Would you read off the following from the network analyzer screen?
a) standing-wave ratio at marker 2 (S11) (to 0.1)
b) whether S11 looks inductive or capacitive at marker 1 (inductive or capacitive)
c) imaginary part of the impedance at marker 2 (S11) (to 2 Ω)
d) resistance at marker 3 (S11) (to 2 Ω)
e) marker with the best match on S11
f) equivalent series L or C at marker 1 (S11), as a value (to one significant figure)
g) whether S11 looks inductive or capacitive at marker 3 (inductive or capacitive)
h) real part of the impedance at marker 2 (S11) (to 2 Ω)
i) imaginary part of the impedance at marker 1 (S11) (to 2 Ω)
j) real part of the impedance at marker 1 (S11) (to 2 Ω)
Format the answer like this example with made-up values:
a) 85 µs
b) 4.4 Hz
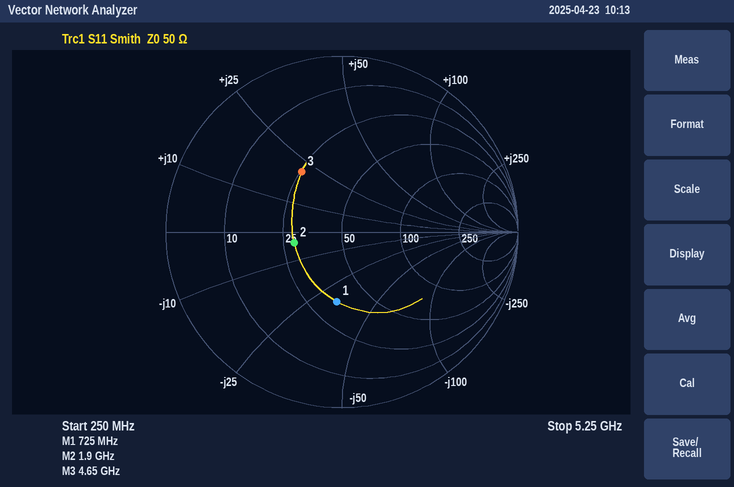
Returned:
a) 1.8
b) capacitive
c) -4 Ω
d) 26 Ω
e) marker 2
f) 7 pF
g) inductive
h) 28 Ω
i) -32 Ω
j) 34 Ω
